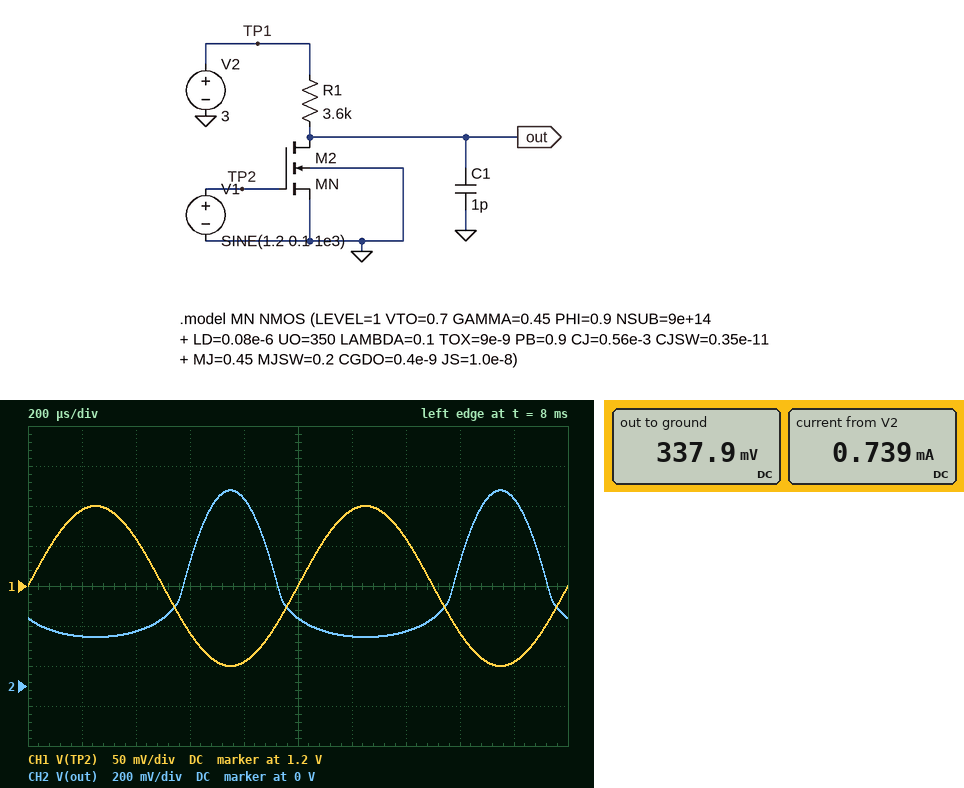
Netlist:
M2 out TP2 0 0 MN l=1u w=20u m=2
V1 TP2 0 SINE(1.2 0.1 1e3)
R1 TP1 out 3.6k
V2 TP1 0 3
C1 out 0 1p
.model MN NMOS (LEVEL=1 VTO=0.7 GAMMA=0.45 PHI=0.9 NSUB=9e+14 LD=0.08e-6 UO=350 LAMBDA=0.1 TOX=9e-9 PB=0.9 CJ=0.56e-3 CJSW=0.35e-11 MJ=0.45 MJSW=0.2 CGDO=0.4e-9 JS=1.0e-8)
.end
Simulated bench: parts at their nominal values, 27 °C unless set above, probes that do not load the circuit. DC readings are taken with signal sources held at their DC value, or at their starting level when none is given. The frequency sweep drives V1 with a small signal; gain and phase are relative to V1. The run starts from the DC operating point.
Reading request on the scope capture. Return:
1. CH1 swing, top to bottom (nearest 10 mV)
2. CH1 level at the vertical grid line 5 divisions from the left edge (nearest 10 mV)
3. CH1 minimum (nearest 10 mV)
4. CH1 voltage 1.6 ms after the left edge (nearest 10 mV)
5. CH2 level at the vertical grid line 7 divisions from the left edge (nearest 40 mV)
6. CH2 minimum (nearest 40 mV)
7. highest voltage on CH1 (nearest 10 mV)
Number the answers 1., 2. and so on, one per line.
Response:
1. 200 mV
2. 1.20 V
3. 1.10 V
4. 1.14 V
5. 280 mV
6. 240 mV
7. 1.30 V
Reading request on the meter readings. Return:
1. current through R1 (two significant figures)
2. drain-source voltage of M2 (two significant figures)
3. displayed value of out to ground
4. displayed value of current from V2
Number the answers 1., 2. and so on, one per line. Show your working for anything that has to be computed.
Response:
1. (3 V - 337.9 mV) / 3.6 kΩ = 740 µA
2. 337.9 mV = 340 mV
3. 337.9 mV
4. 0.739 mA
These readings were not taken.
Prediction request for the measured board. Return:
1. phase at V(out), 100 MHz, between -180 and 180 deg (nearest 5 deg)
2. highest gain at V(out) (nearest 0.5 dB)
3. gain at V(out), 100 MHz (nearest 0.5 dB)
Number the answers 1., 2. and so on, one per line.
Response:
1. 155 deg
2. 4.0 dB
3. 3.0 dB
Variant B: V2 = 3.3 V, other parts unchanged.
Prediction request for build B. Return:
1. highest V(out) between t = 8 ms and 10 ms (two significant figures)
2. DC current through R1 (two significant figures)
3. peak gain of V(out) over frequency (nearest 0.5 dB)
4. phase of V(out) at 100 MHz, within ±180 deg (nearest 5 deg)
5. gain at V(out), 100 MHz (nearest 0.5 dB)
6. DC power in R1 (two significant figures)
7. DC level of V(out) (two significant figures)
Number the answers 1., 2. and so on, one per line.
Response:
1. 1.2 V
2. 800 µA
3. 9.0 dB
4. 145 deg
5. 7.5 dB
6. 2.3 mW
7. 410 mV
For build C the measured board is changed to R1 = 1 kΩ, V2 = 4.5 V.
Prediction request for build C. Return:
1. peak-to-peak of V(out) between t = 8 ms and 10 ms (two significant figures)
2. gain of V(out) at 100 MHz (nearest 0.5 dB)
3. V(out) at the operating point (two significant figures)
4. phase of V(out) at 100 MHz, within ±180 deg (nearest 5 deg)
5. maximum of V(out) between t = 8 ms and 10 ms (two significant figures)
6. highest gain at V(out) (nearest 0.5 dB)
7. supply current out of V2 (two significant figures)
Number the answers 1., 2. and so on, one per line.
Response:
1. 790 mV
2. 10.5 dB
3. 3.4 V
4. 150 deg
5. 3.8 V
6. 12.0 dB
7. 1.1 mA
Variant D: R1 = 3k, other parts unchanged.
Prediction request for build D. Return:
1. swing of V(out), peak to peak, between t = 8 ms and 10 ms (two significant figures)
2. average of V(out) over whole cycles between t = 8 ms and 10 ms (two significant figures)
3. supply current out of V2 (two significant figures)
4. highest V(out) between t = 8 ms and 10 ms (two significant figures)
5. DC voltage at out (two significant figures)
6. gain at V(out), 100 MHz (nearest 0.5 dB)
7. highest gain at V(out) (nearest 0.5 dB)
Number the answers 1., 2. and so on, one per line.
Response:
1. 970 mV
2. 670 mV
3. 840 µA
4. 1.3 V
5. 490 mV
6. 12.0 dB
7. 16.5 dB
